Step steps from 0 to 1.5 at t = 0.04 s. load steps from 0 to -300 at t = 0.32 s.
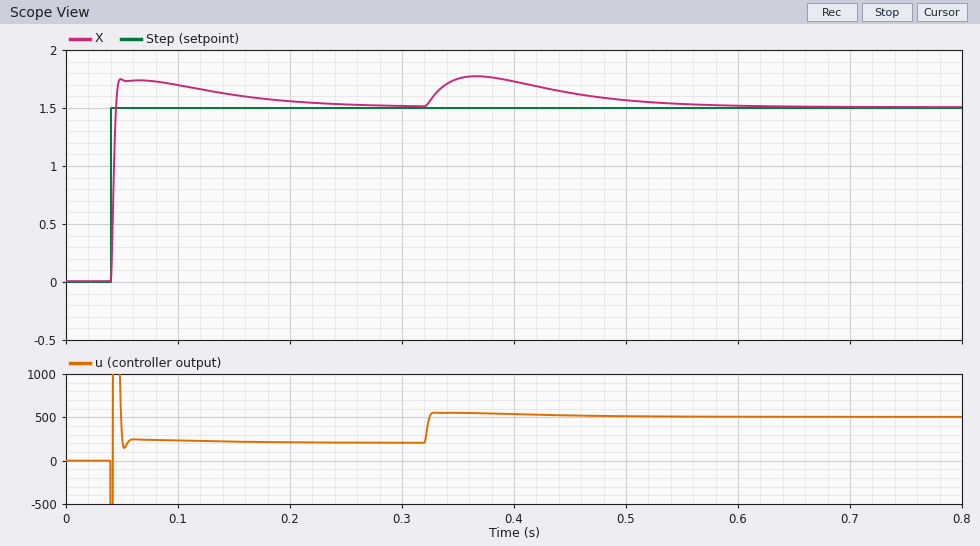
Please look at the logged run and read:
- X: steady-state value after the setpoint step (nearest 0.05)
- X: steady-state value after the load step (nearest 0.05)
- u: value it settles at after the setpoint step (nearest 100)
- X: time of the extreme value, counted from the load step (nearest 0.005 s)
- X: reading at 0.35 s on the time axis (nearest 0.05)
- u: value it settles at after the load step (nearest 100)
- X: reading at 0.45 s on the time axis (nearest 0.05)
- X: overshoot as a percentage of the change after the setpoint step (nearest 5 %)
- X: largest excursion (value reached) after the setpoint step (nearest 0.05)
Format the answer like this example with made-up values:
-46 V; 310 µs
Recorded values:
1.50; 1.50; 200; 0.045 s; 1.75; 500; 1.65; 15 %; 1.75
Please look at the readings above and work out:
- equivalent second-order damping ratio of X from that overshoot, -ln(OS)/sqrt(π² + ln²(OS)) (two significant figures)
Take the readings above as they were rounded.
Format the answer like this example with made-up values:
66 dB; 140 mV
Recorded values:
0.52
